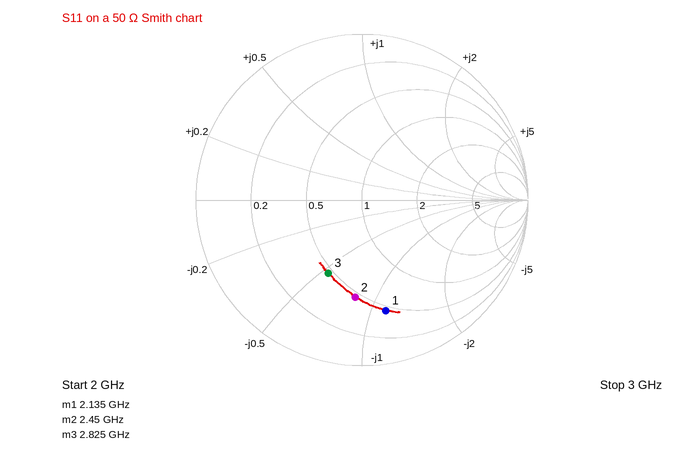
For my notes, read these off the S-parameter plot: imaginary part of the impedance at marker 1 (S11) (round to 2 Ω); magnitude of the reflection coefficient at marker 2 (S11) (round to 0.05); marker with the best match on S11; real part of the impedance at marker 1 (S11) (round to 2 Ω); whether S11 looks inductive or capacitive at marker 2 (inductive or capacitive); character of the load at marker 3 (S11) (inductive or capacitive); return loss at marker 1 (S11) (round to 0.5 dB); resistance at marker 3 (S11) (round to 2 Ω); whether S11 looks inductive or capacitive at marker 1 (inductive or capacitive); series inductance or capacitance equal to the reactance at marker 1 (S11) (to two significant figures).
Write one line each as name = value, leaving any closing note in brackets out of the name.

imaginary part of the impedance at marker 1 (S11) = -56 Ω
magnitude of the reflection coefficient at marker 2 (S11) = 0.60
marker with the best match on S11 = marker 3
real part of the impedance at marker 1 (S11) = 22 Ω
whether S11 looks inductive or capacitive at marker 2 = capacitive
character of the load at marker 3 (S11) = capacitive
return loss at marker 1 (S11) = 3.5 dB
resistance at marker 3 (S11) = 24 Ω
whether S11 looks inductive or capacitive at marker 1 = capacitive
series inductance or capacitance equal to the reactance at marker 1 (S11) = 1.3 pF
